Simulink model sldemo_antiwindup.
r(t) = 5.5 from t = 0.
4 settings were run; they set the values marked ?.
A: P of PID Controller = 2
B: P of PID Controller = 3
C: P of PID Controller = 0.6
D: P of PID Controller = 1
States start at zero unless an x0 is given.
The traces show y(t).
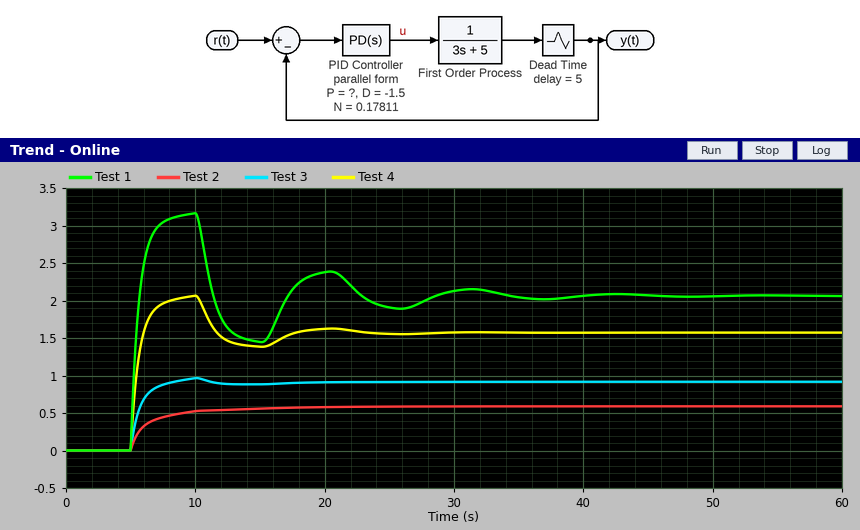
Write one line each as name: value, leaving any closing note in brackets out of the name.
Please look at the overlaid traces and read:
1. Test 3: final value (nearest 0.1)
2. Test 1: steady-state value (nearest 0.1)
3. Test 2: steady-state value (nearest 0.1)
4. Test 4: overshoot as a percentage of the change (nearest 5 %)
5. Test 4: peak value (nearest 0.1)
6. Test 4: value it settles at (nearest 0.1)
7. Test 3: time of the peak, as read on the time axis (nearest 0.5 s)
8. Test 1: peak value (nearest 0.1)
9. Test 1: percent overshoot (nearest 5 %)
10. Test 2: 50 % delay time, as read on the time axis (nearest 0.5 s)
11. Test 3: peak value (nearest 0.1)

Test 3: final value: 0.9
Test 1: steady-state value: 2.1
Test 2: steady-state value: 0.6
Test 4: overshoot as a percentage of the change: 30 %
Test 4: peak value: 2.1
Test 4: value it settles at: 1.6
Test 3: time of the peak, as read on the time axis: 10.0 s
Test 1: peak value: 3.2
Test 1: percent overshoot: 55 %
Test 2: 50 % delay time, as read on the time axis: 6.0 s
Test 3: peak value: 1.0
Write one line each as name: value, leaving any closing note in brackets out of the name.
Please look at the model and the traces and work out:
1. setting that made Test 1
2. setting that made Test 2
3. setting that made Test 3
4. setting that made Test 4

setting that made Test 1: B
setting that made Test 2: C
setting that made Test 3: D
setting that made Test 4: A
